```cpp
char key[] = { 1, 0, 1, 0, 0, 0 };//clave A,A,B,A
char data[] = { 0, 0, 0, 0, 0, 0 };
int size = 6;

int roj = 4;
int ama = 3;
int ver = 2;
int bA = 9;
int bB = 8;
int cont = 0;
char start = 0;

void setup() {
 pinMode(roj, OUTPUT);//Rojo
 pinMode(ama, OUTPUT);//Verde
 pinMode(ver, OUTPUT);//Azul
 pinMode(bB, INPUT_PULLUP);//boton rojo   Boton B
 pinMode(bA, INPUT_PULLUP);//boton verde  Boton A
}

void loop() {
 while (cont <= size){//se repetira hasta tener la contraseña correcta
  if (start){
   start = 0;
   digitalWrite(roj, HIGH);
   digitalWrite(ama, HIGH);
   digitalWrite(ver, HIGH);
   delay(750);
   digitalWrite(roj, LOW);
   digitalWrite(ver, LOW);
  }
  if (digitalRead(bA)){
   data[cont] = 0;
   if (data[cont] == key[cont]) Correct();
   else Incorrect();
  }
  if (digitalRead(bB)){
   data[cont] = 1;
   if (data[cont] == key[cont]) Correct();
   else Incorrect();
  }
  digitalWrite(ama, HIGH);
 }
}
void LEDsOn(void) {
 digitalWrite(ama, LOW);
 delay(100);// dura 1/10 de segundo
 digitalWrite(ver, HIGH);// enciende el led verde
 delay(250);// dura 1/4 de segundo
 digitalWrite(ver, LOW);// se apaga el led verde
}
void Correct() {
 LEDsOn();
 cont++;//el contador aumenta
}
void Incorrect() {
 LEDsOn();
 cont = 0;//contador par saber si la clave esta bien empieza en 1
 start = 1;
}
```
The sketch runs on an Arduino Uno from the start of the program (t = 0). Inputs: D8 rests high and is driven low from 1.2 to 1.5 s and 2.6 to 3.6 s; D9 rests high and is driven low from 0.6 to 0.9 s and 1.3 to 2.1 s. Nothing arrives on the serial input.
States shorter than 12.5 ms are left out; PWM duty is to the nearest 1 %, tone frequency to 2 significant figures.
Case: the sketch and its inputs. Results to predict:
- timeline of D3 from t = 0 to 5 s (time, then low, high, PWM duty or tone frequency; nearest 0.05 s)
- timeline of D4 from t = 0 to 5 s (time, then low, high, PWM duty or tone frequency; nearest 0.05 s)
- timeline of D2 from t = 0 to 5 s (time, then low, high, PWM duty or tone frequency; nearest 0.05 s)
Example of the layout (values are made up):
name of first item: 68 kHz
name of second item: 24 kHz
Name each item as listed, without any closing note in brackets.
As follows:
timeline of D3 from t = 0 to 5 s: 0 s low; 0.7 s high; 1.5 s low; 1.85 s high; 2.6 s low; 2.95 s high; 3.7 s low; 4.4 s high
timeline of D4 from t = 0 to 5 s: 0 s low; 0.7 s high; 1.45 s low; 1.85 s high; 2.6 s low; 2.95 s high; 3.7 s low; 4.4 s high
timeline of D2 from t = 0 to 5 s: 0 s low; 0.1 s high; 0.35 s low; 0.45 s high; 1.45 s low; 1.6 s high; 2.6 s low; 2.7 s high; 3.7 s low; 3.8 s high; 4.05 s low; 4.15 s high
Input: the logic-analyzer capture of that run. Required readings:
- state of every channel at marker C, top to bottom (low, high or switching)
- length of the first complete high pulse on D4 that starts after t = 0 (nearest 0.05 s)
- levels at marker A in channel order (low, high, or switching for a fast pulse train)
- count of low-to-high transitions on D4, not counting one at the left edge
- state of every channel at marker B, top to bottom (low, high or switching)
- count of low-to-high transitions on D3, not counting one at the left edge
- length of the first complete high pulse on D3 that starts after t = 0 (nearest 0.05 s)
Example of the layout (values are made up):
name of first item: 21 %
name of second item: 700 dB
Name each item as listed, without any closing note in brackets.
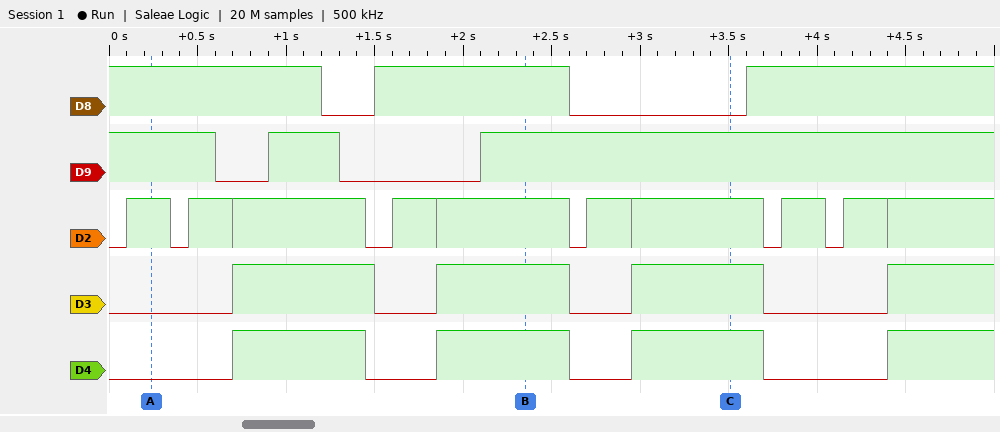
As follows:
state of every channel at marker C, top to bottom: D8 low, D9 high, D2 high, D3 high, D4 high
length of the first complete high pulse on D4 that starts after t = 0: 0.75 s
levels at marker A in channel order: D8 high, D9 high, D2 high, D3 low, D4 low
count of low-to-high transitions on D4, not counting one at the left edge: 4
state of every channel at marker B, top to bottom: D8 high, D9 high, D2 high, D3 high, D4 high
count of low-to-high transitions on D3, not counting one at the left edge: 4
length of the first complete high pulse on D3 that starts after t = 0: 0.80 s
